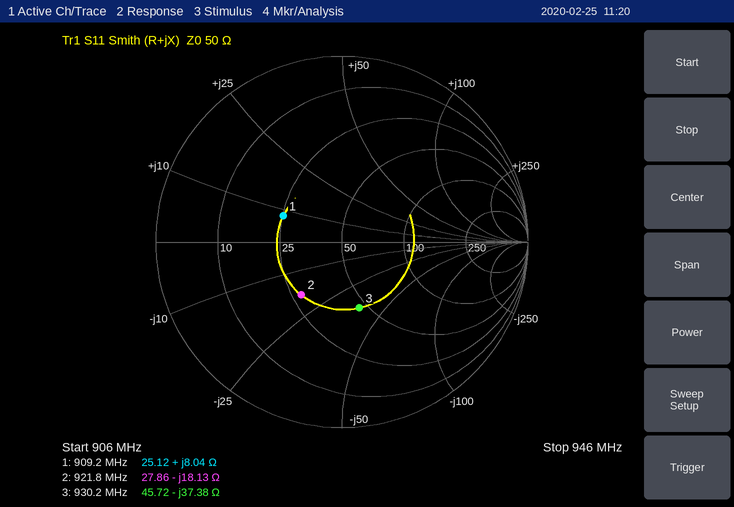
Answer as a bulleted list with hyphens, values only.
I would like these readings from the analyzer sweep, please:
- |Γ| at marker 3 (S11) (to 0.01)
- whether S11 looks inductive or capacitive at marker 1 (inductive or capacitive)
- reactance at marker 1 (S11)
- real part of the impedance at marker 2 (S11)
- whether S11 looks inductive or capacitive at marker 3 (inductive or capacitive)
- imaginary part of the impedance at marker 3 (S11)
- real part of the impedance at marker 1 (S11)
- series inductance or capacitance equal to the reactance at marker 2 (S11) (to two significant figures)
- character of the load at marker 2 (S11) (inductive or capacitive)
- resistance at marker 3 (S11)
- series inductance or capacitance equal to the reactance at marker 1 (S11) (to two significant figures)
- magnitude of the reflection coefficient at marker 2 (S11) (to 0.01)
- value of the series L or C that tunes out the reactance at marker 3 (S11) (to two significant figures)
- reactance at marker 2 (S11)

- 0.37
- inductive
- +8.04 Ω
- 27.86 Ω
- capacitive
- -37.38 Ω
- 25.12 Ω
- 9.5 pF
- capacitive
- 45.72 Ω
- 1.4 nH
- 0.36
- 6.4 nH
- -18.13 Ω
